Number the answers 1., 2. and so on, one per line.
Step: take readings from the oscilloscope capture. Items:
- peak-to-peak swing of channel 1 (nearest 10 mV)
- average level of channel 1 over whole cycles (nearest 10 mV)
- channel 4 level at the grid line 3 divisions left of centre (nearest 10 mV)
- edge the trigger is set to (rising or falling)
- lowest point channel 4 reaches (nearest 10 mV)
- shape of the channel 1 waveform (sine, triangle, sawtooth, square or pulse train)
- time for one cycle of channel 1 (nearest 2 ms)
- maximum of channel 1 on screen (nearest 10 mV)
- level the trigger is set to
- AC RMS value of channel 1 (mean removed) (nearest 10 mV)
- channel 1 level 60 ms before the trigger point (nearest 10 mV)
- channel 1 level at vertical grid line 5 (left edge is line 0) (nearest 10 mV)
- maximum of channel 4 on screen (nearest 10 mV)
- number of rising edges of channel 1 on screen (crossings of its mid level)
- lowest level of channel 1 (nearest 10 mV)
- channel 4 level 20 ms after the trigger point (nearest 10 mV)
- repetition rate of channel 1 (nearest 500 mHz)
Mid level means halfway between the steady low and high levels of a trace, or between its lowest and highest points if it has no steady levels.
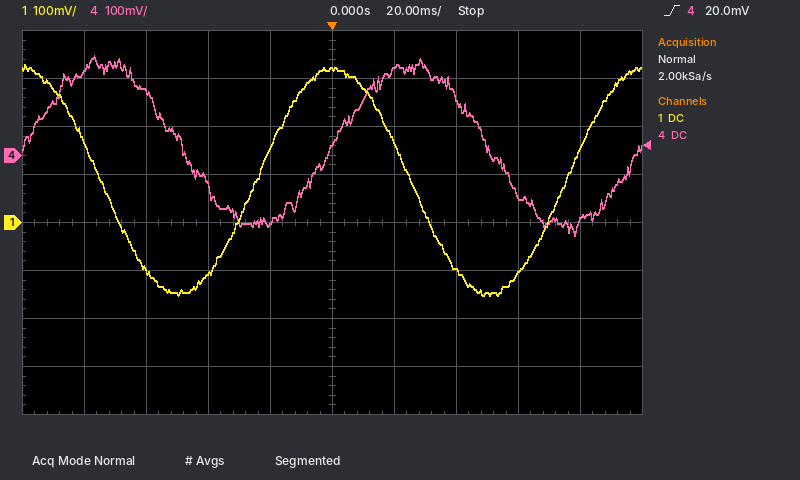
1. 480 mV
2. 90 mV
3. 130 mV
4. rising
5. -170 mV
6. sine
7. 100 ms
8. 330 mV
9. 20.0 mV
10. 170 mV
11. -100 mV
12. 320 mV
13. 210 mV
14. 2
15. -150 mV
16. 180 mV
17. 10.0 Hz
